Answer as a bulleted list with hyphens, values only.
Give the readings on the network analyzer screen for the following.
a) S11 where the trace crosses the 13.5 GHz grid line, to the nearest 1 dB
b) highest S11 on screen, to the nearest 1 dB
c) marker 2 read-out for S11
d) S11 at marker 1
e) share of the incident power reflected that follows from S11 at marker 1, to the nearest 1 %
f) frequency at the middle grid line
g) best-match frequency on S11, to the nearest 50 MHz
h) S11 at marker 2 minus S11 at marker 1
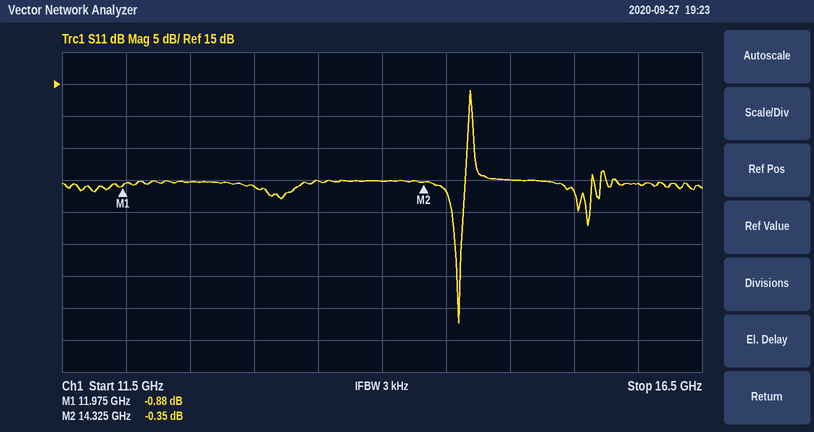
- 0 dB
- 14 dB
- -0.35 dB
- -0.88 dB
- 82 %
- 14 GHz
- 14.60 GHz
- 0.53 dB
